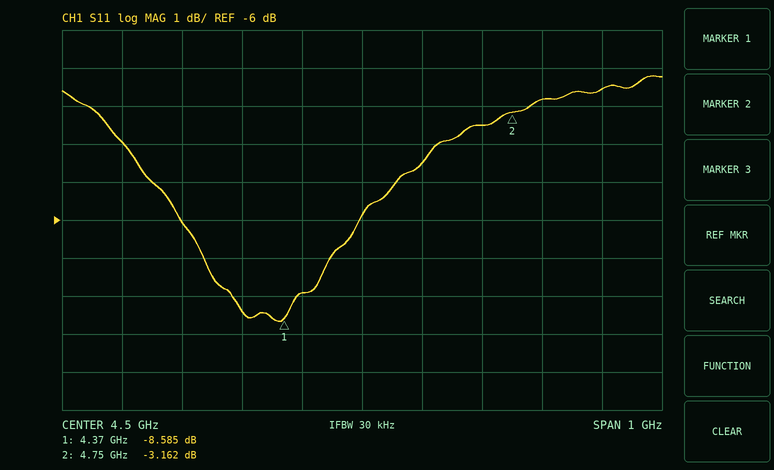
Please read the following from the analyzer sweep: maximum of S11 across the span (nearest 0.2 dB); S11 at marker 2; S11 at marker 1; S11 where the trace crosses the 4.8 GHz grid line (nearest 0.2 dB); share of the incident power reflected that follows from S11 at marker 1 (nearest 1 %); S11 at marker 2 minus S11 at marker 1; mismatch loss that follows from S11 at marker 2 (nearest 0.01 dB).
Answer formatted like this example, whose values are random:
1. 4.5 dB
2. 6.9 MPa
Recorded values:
1. -2.2 dB
2. -3.162 dB
3. -8.585 dB
4. -2.8 dB
5. 14 %
6. 5.423 dB
7. 2.86 dB
